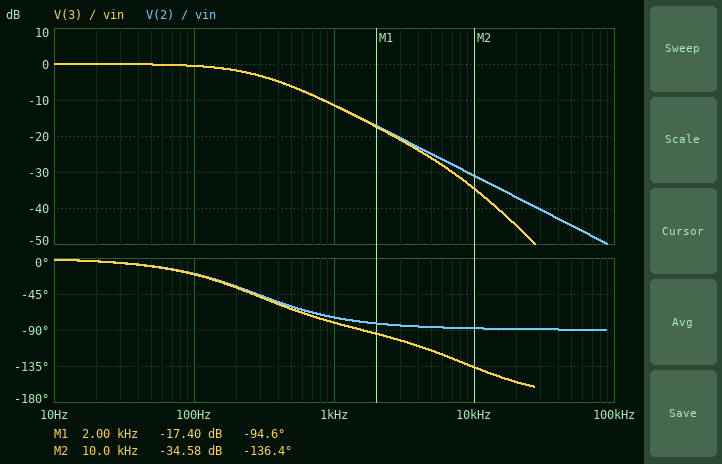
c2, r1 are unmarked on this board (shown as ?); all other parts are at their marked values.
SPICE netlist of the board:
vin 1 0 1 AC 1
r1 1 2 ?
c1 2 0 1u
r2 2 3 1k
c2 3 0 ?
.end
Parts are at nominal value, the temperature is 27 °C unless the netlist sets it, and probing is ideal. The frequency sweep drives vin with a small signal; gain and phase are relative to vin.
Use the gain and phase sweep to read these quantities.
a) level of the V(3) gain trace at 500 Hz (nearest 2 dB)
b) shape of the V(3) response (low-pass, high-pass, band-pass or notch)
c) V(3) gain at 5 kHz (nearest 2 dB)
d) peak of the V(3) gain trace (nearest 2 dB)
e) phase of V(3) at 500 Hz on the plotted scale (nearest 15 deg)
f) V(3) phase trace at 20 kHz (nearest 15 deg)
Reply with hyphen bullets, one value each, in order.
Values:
- -6 dB
- low-pass
- -26 dB
- 0 dB
- -60 deg
- -150 deg
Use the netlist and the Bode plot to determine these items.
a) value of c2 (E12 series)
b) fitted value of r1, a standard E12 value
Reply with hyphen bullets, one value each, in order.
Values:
- 18 nF
- 560 Ω
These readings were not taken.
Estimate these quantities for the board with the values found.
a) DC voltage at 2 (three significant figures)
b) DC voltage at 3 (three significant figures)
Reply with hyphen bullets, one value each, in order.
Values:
- 1.00 V
- 1.00 V
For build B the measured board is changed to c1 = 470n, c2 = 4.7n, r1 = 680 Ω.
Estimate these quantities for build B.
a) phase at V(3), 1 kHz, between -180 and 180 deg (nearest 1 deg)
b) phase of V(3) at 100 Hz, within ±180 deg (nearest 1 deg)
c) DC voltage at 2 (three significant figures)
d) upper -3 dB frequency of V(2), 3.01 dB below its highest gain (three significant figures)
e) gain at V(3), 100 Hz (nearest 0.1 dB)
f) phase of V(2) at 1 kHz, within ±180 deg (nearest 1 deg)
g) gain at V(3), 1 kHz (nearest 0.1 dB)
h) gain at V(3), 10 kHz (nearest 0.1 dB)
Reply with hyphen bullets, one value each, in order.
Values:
- -65 deg
- -12 deg
- 1.00 V
- 493 Hz
- -0.2 dB
- -64 deg
- -7.1 dB
- -26.5 dB
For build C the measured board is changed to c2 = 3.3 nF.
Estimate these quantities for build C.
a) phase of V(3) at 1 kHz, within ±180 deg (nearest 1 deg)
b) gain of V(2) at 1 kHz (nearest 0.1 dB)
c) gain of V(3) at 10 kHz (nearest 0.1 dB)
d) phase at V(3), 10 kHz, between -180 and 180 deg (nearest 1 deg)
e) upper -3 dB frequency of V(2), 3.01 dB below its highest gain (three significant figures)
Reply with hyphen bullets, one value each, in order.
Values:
- -75 deg
- -11.3 dB
- -31.1 dB
- -100 deg
- 283 Hz
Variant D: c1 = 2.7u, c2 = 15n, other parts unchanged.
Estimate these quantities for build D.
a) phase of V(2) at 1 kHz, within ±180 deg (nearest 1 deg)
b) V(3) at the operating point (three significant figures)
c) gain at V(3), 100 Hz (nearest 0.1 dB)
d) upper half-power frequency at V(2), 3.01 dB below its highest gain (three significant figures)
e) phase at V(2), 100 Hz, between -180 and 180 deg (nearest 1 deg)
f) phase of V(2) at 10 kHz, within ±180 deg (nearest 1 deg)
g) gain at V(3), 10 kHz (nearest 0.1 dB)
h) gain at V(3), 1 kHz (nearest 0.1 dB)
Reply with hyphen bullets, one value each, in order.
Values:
- -84 deg
- 1.00 V
- -2.8 dB
- 105 Hz
- -44 deg
- -89 deg
- -42.3 dB
- -19.7 dB
